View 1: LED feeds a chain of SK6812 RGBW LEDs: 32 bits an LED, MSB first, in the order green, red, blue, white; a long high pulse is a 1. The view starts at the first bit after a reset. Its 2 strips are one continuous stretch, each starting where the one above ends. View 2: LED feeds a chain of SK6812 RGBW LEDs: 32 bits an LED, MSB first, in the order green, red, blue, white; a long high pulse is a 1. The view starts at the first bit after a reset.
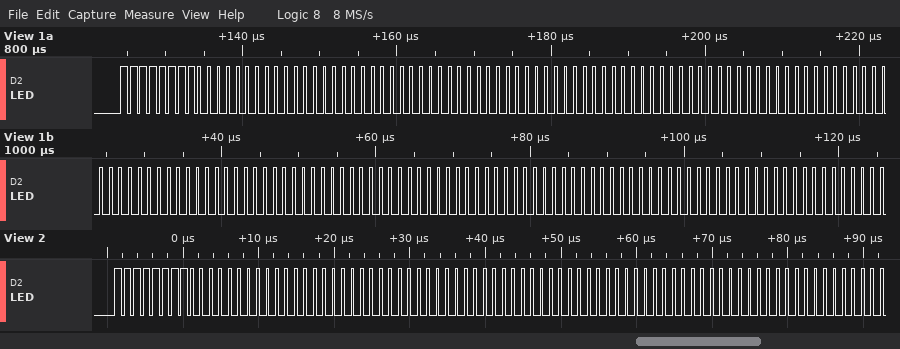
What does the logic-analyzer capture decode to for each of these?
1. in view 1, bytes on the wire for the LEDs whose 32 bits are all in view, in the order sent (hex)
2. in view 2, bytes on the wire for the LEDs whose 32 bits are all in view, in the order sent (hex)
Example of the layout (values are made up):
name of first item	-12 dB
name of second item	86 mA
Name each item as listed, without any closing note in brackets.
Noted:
in view 1, bytes on the wire for the LEDs whose 32 bits are all in view, in the order sent	FF 00 00 00 00 00 00 00 00 00 00 00 00 00 00 00 00 00 00 00
in view 2, bytes on the wire for the LEDs whose 32 bits are all in view, in the order sent	FF 00 00 00 00 00 00 00
